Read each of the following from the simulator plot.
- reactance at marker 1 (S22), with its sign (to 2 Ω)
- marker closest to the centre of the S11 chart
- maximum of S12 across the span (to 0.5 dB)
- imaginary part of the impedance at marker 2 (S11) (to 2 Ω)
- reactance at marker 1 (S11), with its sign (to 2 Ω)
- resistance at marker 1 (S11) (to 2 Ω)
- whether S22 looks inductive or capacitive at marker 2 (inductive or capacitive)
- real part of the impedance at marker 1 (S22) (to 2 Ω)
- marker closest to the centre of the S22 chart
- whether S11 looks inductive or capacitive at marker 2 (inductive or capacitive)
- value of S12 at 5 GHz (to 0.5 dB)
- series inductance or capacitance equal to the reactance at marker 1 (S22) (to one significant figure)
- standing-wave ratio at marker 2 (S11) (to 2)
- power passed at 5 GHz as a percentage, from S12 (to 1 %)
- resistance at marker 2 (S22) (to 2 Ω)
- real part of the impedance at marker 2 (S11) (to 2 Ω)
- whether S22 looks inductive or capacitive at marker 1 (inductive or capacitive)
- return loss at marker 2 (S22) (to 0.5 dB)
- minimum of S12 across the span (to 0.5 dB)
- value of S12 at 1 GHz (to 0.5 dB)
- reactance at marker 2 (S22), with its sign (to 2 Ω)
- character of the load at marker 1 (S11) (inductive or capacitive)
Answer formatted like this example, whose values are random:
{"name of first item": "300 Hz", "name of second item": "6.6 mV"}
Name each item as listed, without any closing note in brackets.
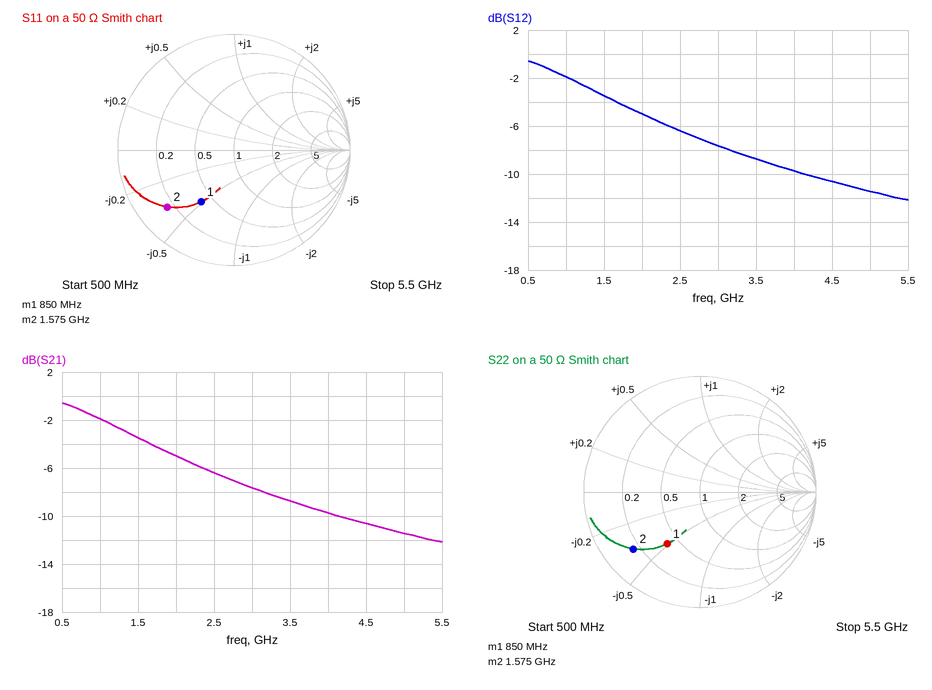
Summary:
{"reactance at marker 1 (S22), with its sign": "-24 Ω", "marker closest to the centre of the S11 chart": "marker 1", "maximum of S12 across the span": "-0.5 dB", "imaginary part of the impedance at marker 2 (S11)": "-18 Ω", "reactance at marker 1 (S11), with its sign": "-24 Ω", "resistance at marker 1 (S11)": "20 Ω", "whether S22 looks inductive or capacitive at marker 2": "capacitive", "real part of the impedance at marker 1 (S22)": "20 Ω", "marker closest to the centre of the S22 chart": "marker 1", "whether S11 looks inductive or capacitive at marker 2": "capacitive", "value of S12 at 5 GHz": "-11.5 dB", "series inductance or capacitance equal to the reactance at marker 1 (S22)": "8 pF", "standing-wave ratio at marker 2 (S11)": "8", "power passed at 5 GHz as a percentage, from S12": "7 %", "resistance at marker 2 (S22)": "8 Ω", "real part of the impedance at marker 2 (S11)": "8 Ω", "whether S22 looks inductive or capacitive at marker 1": "capacitive", "return loss at marker 2 (S22)": "2.5 dB", "minimum of S12 across the span": "-12.0 dB", "value of S12 at 1 GHz": "-2.0 dB", "reactance at marker 2 (S22), with its sign": "-18 Ω", "character of the load at marker 1 (S11)": "capacitive"}
